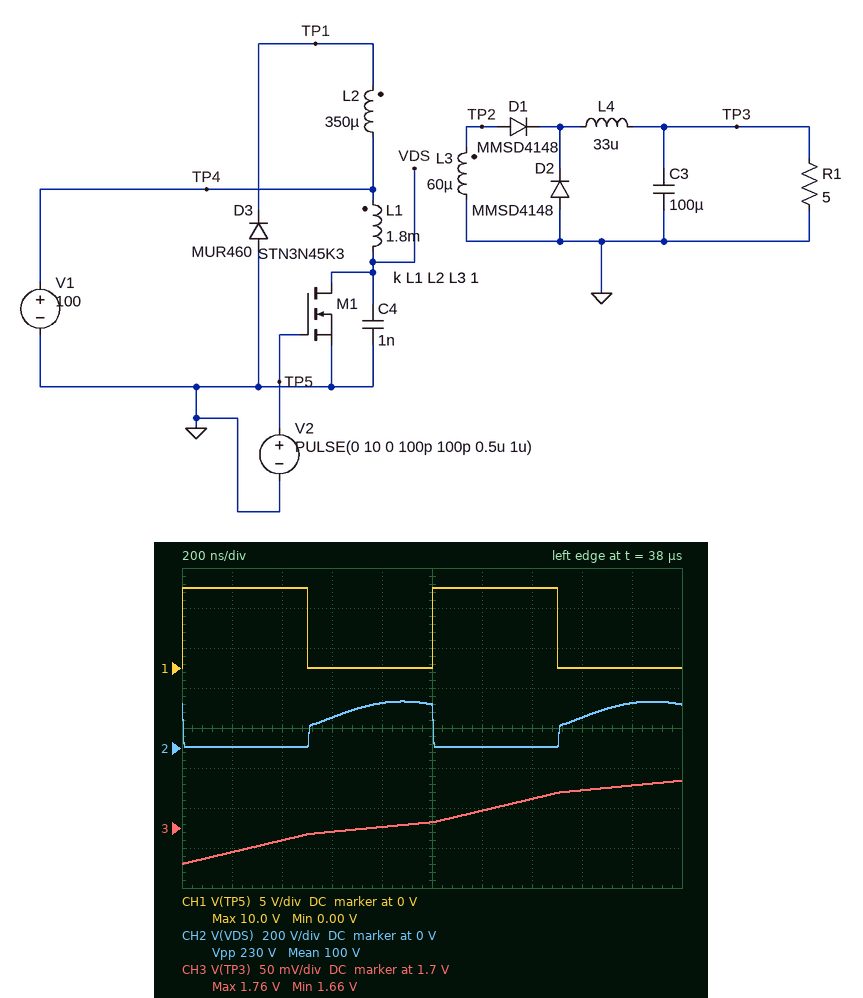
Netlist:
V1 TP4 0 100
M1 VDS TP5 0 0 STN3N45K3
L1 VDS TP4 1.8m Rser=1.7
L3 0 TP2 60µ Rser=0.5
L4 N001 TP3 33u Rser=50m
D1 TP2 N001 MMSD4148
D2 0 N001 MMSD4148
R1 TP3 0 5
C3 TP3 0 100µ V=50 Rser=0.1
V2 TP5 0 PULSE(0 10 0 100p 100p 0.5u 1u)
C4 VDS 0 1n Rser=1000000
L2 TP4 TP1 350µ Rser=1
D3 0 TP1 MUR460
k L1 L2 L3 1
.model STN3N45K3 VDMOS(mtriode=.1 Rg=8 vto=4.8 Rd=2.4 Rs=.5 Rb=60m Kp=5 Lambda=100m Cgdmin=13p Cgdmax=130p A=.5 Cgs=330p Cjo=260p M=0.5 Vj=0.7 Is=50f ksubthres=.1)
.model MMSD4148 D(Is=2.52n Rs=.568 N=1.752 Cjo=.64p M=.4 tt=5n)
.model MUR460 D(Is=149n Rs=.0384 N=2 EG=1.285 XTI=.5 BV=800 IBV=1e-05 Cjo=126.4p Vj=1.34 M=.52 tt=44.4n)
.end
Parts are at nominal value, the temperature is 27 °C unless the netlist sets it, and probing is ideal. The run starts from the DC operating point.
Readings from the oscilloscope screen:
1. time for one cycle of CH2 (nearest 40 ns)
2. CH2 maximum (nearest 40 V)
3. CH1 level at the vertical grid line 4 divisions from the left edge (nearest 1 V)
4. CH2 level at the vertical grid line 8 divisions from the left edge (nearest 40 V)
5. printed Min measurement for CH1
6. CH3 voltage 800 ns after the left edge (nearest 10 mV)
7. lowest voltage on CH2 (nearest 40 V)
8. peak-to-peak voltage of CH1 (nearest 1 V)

1.00 µs
240 V
0 V
160 V
0.00 V
1.70 V
0 V
10 V
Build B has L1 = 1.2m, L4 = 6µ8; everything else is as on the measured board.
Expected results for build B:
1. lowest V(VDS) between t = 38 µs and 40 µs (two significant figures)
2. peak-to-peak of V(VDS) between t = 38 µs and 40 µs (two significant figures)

5.2 V
220 V
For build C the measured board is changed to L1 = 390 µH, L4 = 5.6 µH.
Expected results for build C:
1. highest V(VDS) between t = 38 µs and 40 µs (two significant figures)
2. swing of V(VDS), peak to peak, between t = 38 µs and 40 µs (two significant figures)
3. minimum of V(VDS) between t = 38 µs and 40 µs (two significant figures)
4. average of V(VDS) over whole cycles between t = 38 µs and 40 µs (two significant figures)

210 V
190 V
14 V
96 V
